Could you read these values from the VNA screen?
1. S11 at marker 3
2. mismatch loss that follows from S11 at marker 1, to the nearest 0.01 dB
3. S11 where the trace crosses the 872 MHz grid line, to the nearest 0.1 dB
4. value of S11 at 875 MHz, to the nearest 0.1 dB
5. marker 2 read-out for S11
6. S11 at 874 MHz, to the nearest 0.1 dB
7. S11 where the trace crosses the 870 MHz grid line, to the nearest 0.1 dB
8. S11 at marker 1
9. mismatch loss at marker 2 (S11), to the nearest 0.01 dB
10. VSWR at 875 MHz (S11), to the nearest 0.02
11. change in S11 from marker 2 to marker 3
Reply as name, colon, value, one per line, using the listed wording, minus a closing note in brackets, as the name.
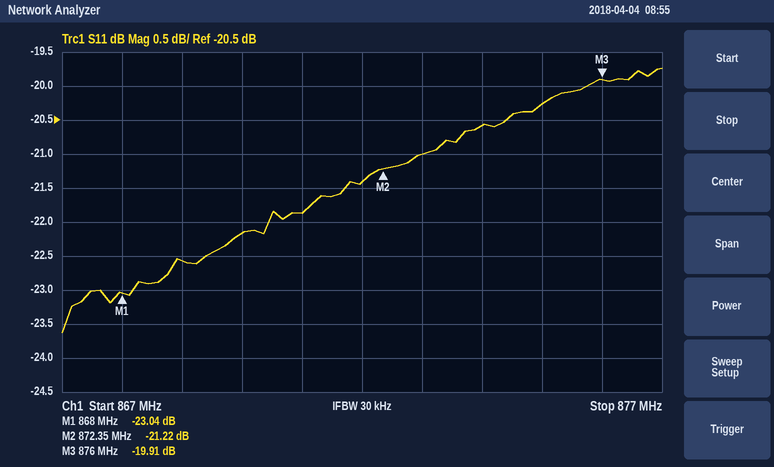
S11 at marker 3: -19.91 dB
mismatch loss that follows from S11 at marker 1, to the nearest 0.01 dB: 0.02 dB
S11 where the trace crosses the 872 MHz grid line, to the nearest 0.1 dB: -21.4 dB
value of S11 at 875 MHz, to the nearest 0.1 dB: -20.3 dB
marker 2 read-out for S11: -21.22 dB
S11 at 874 MHz, to the nearest 0.1 dB: -20.6 dB
S11 where the trace crosses the 870 MHz grid line, to the nearest 0.1 dB: -22.2 dB
S11 at marker 1: -23.04 dB
mismatch loss at marker 2 (S11), to the nearest 0.01 dB: 0.03 dB
VSWR at 875 MHz (S11), to the nearest 0.02: 1.22
change in S11 from marker 2 to marker 3: 1.31 dB
